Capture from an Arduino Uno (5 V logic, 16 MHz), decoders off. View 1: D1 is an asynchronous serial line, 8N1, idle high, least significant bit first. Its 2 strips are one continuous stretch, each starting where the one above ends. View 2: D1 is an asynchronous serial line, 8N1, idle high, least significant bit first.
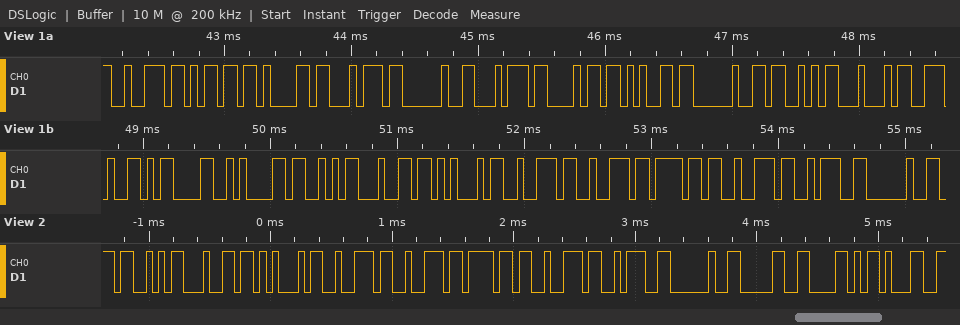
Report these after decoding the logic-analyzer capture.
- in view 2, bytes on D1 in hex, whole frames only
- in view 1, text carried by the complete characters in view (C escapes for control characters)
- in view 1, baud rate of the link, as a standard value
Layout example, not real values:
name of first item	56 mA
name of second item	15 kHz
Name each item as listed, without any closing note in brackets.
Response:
in view 2, bytes on D1 in hex, whole frames only	0x53 0x64 0x45 0x72 0x72 0x6F 0x72 0x3A 0x20 0x30 0x58 0x31
in view 1, text carried by the complete characters in view	"rmat the SD.\r\nSdError: "
in view 1, baud rate of the link, as a standard value	19200 baud
